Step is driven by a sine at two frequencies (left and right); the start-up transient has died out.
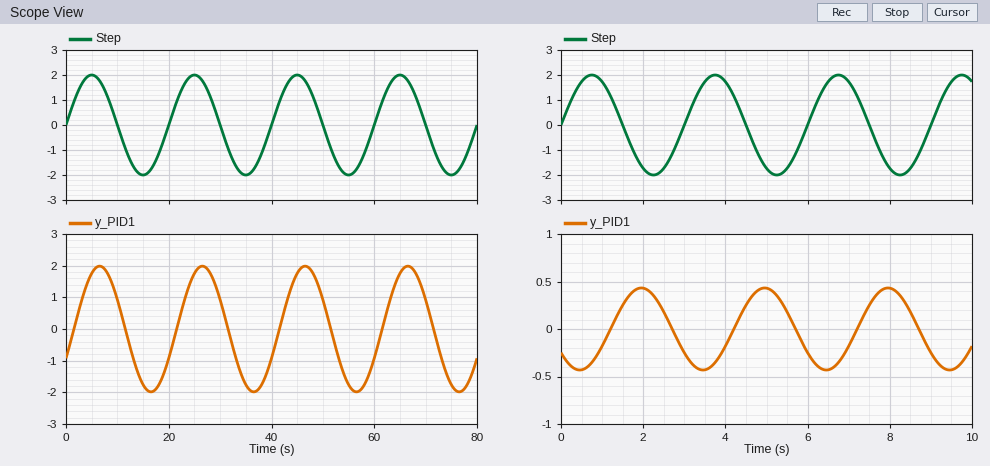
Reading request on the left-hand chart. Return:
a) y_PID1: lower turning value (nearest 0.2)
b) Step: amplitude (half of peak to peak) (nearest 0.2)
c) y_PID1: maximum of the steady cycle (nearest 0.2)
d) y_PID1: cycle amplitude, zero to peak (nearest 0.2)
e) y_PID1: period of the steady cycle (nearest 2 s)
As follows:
-2.0
2.0
2.0
2.0
20 s
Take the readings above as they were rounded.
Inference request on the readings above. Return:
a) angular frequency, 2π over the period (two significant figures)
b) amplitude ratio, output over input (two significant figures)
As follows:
0.31 rad/s
1.0
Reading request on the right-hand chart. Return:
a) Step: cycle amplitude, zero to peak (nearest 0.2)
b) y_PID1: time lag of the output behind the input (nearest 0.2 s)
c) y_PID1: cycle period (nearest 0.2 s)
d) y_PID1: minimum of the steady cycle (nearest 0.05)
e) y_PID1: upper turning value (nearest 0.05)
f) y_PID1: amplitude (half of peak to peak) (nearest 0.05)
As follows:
2.0
1.2 s
3.0 s
-0.45
0.45
0.45
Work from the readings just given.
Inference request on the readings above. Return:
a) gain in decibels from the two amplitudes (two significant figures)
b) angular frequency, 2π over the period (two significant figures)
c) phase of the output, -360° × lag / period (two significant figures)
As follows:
-13 dB
2.1 rad/s
-140°
